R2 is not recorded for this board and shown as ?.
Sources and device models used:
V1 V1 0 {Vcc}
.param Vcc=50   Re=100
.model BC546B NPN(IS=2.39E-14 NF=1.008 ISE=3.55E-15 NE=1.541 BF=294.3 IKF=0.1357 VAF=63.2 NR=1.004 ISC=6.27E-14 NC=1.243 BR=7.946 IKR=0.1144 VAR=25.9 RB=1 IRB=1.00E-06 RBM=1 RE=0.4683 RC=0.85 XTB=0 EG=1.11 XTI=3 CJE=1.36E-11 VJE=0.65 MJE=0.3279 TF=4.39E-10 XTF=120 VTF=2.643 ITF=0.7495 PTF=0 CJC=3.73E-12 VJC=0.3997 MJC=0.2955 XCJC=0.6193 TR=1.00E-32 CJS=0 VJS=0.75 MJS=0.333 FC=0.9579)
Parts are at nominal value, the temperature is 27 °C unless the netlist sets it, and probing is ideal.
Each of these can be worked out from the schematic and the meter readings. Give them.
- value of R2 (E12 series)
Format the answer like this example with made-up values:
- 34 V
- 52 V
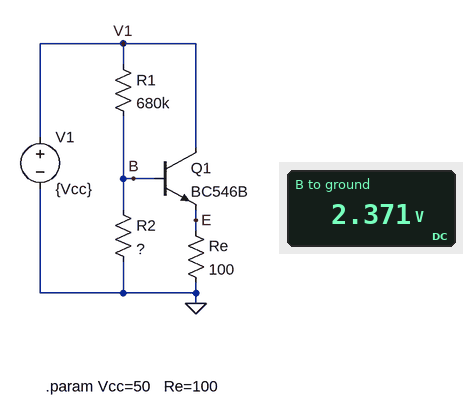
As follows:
- 68 kΩ
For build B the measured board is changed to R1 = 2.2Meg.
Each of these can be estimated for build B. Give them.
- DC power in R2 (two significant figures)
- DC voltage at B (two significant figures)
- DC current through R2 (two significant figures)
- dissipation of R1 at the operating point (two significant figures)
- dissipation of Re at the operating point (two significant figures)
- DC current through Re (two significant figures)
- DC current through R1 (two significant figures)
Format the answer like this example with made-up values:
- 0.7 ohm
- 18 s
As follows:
- 15 µW
- 1.0 V
- 15 µA
- 1.1 mW
- 1.3 mW
- 3.6 mA
- 22 µA
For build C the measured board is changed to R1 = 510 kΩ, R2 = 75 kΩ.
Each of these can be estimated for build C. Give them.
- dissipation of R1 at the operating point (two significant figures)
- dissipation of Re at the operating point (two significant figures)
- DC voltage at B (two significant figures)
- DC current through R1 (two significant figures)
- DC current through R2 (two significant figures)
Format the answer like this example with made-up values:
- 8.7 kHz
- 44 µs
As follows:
- 4.3 mW
- 55 mW
- 3.1 V
- 92 µA
- 41 µA
